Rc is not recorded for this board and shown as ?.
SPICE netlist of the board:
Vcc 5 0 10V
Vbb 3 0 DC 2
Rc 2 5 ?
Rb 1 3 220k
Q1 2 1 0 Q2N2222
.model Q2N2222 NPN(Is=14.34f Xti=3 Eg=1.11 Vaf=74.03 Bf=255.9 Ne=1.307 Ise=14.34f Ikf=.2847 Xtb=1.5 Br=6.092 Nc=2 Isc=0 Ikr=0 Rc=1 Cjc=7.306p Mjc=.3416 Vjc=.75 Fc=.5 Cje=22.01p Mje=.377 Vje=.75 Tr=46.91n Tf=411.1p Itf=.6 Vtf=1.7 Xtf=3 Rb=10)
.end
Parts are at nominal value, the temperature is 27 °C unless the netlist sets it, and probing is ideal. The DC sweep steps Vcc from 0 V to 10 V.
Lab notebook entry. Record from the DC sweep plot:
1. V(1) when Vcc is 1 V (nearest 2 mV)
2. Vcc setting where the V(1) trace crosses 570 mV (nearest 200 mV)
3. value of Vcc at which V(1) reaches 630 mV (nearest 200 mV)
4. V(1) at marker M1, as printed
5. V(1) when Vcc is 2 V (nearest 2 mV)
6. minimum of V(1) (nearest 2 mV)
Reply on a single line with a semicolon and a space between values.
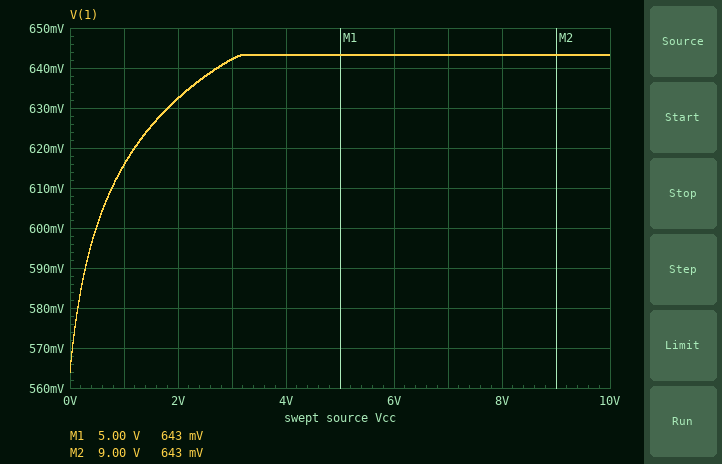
616 mV; 0 V; 1.8 V; 643 mV; 632 mV; 564 mV
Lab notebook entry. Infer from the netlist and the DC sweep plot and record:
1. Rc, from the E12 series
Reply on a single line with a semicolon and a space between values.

3.3 kΩ
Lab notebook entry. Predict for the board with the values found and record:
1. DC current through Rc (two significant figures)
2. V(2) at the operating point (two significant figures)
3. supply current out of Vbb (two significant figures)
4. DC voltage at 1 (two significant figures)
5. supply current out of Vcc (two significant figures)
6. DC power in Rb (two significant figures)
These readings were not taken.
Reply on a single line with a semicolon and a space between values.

980 µA; 6.8 V; 6.2 µA; 640 mV; 980 µA; 8.4 µW
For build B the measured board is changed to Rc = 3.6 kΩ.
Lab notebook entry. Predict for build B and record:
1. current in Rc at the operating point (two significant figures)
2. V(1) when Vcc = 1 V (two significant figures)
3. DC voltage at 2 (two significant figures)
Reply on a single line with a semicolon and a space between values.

970 µA; 610 mV; 6.5 V
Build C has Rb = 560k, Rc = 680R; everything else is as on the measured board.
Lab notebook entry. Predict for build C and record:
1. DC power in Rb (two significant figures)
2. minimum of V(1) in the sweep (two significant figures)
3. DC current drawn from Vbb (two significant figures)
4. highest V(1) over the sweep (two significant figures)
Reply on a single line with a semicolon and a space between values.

3.4 µW; 540 mV; 2.5 µA; 620 mV
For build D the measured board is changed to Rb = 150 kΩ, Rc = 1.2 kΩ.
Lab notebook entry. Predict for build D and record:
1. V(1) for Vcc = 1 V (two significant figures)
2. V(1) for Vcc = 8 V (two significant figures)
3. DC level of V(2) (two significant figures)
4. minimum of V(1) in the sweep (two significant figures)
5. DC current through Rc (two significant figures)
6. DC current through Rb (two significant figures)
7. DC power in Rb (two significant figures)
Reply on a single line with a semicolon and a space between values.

640 mV; 650 mV; 8.2 V; 570 mV; 1.5 mA; 9.0 µA; 12 µW
